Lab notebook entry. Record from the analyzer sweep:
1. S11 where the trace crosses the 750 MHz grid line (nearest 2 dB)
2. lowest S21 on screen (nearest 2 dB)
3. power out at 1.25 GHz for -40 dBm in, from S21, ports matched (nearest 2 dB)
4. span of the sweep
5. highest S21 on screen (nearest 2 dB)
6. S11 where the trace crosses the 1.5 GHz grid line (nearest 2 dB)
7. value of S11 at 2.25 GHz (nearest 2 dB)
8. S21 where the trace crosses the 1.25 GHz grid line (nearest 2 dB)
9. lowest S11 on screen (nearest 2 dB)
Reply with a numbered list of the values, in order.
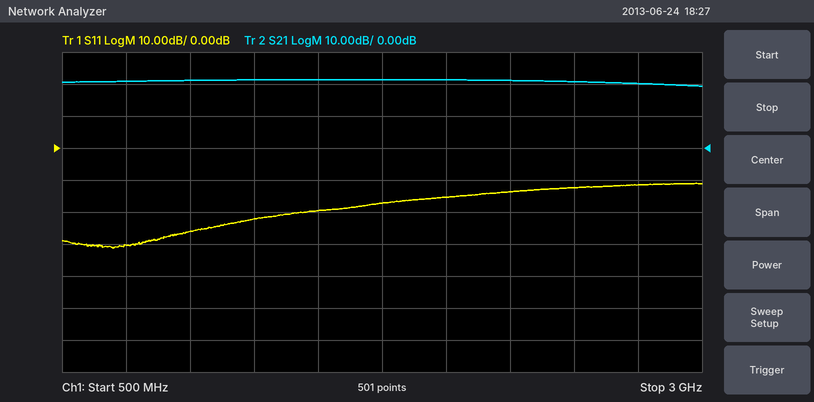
1. -30 dB
2. 20 dB
3. -18 dBm
4. 2.5 GHz
5. 22 dB
6. -20 dB
7. -14 dB
8. 22 dB
9. -32 dB
